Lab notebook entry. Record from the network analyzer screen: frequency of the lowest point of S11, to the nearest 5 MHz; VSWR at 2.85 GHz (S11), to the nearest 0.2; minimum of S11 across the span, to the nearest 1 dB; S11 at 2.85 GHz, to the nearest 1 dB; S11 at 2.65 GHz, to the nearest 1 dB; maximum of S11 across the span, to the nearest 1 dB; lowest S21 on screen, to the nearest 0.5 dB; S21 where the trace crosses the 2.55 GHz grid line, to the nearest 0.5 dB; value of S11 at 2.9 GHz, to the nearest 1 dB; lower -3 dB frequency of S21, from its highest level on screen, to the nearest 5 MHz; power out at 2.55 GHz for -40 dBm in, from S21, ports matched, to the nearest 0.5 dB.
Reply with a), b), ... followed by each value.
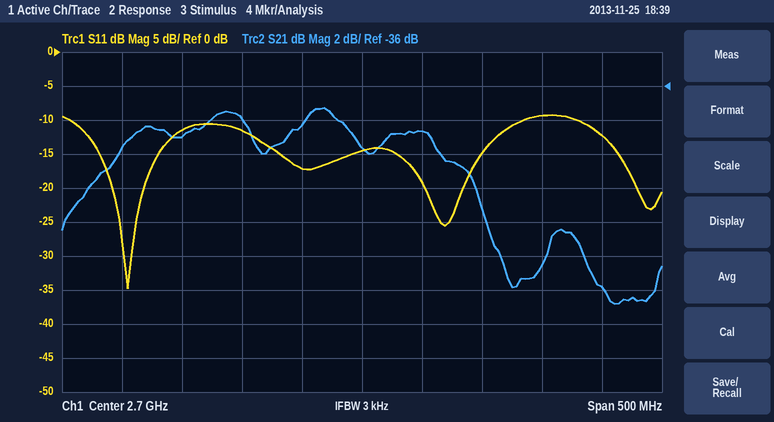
a) 2.505 GHz
b) 2.0
c) -35 dB
d) -9 dB
e) -17 dB
f) -9 dB
g) -49.0 dB
h) -39.0 dB
i) -12 dB
j) 2.495 GHz
k) -79.0 dBm
